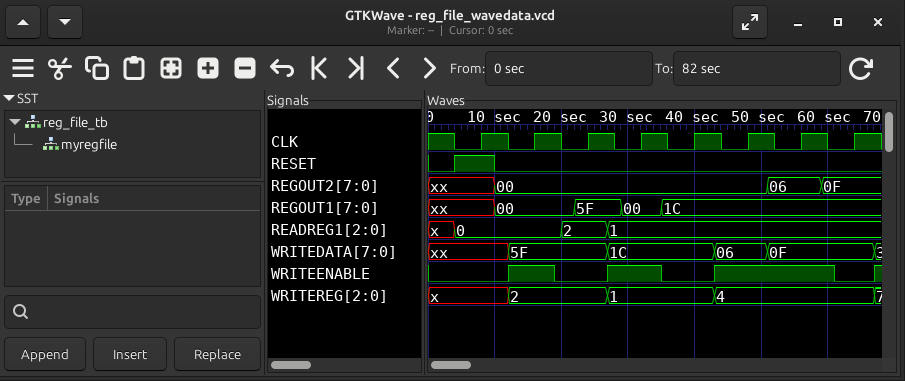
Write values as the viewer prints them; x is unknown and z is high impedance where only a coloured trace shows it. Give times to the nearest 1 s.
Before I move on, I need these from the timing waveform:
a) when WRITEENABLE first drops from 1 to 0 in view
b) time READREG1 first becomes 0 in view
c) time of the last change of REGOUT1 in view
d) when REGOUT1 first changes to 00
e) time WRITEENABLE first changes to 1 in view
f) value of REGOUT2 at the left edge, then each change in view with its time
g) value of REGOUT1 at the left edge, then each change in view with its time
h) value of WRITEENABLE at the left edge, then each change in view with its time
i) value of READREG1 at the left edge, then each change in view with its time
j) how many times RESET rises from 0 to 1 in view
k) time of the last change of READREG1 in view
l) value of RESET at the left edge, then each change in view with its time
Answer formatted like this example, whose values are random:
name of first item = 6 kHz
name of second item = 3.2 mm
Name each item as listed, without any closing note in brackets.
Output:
when WRITEENABLE first drops from 1 to 0 in view = 19 s
time READREG1 first becomes 0 in view = 4 s
time of the last change of REGOUT1 in view = 35 s
when REGOUT1 first changes to 00 = 10 s
time WRITEENABLE first changes to 1 in view = 12 s
value of REGOUT2 at the left edge, then each change in view with its time = xx, 00 at 10 s, 06 at 51 s, 0F at 59 s
value of REGOUT1 at the left edge, then each change in view with its time = xx, 00 at 10 s, 5F at 22 s, 00 at 29 s, 1C at 35 s
value of WRITEENABLE at the left edge, then each change in view with its time = 0, 1 at 12 s, 0 at 19 s, 1 at 27 s, 0 at 35 s, 1 at 43 s, 0 at 61 s, 1 at 67 s
value of READREG1 at the left edge, then each change in view with its time = x, 0 at 4 s, 2 at 20 s, 1 at 27 s
how many times RESET rises from 0 to 1 in view = 1
time of the last change of READREG1 in view = 27 s
value of RESET at the left edge, then each change in view with its time = 0, 1 at 4 s, 0 at 10 s
